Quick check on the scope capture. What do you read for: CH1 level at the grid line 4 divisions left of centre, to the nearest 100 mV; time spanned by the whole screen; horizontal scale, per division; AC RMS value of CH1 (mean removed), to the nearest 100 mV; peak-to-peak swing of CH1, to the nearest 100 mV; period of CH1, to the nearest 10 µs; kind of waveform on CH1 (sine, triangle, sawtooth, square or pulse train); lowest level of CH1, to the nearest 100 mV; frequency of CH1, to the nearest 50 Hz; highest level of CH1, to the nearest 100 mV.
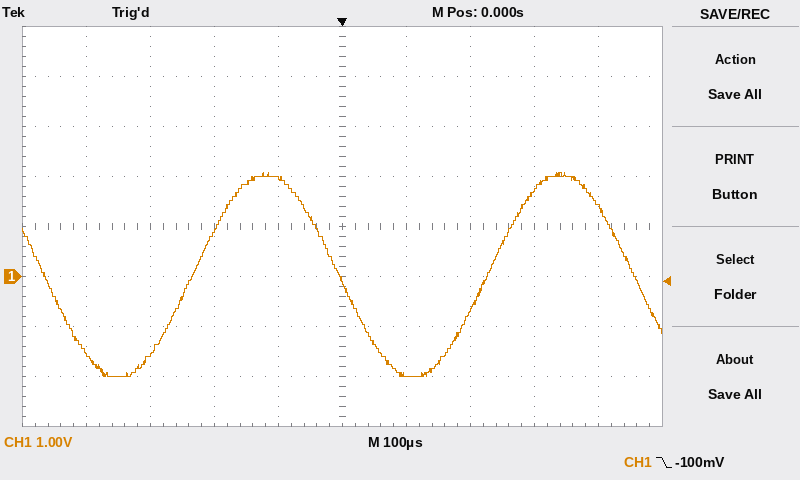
-1.5 V
1 ms
100 µs
1.4 V
4.1 V
460 µs
sine
-2.0 V
2.15 kHz
2.1 V
